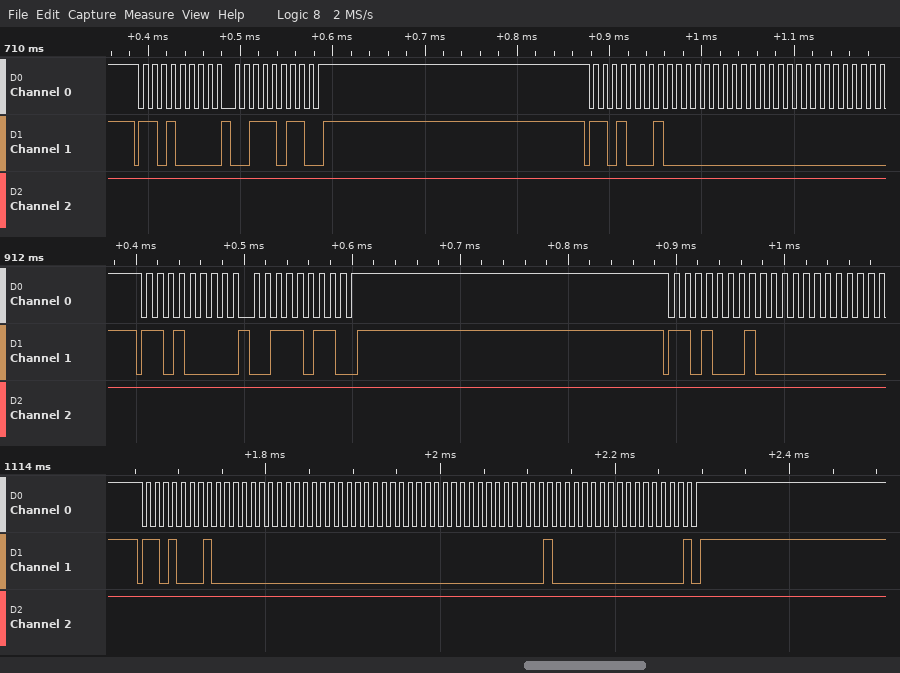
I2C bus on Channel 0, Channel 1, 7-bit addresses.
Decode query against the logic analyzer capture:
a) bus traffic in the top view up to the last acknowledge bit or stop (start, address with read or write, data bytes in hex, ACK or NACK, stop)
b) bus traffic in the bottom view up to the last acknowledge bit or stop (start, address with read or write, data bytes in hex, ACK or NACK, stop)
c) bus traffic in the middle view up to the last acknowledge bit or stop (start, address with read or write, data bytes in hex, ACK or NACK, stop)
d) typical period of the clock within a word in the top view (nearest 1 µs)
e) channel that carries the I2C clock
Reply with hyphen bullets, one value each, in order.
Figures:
- start, address 68 write ACK, 3B ACK, stop, start, address 68 read ACK, 00 ACK, 00 ACK
- start, address 68 read ACK, 00 ACK, 00 ACK, 00 ACK, 00 ACK, 40 ACK, 00 NACK, stop
- start, address 68 write ACK, 3B ACK, stop, start, address 68 read ACK, 00 ACK
- 10 µs
- Channel 0
